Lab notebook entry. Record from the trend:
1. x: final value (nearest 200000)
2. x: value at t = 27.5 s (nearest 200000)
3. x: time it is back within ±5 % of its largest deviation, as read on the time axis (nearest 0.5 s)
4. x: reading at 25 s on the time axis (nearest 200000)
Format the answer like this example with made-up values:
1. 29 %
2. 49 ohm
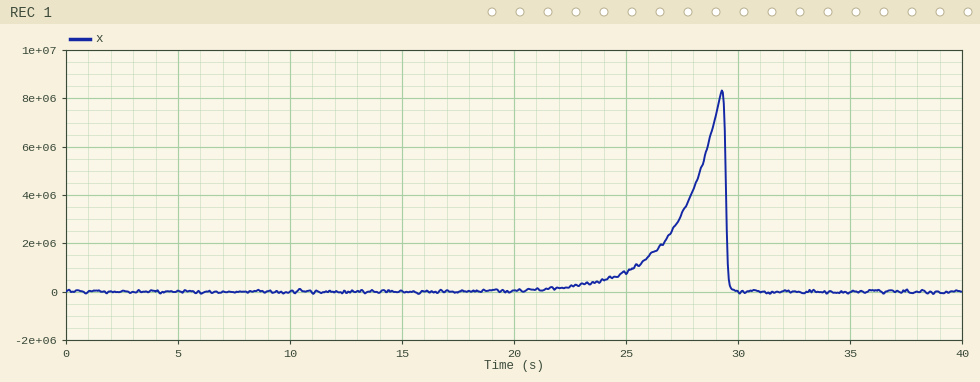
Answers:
1. 0
2. 3200000
3. 29.5 s
4. 800000
